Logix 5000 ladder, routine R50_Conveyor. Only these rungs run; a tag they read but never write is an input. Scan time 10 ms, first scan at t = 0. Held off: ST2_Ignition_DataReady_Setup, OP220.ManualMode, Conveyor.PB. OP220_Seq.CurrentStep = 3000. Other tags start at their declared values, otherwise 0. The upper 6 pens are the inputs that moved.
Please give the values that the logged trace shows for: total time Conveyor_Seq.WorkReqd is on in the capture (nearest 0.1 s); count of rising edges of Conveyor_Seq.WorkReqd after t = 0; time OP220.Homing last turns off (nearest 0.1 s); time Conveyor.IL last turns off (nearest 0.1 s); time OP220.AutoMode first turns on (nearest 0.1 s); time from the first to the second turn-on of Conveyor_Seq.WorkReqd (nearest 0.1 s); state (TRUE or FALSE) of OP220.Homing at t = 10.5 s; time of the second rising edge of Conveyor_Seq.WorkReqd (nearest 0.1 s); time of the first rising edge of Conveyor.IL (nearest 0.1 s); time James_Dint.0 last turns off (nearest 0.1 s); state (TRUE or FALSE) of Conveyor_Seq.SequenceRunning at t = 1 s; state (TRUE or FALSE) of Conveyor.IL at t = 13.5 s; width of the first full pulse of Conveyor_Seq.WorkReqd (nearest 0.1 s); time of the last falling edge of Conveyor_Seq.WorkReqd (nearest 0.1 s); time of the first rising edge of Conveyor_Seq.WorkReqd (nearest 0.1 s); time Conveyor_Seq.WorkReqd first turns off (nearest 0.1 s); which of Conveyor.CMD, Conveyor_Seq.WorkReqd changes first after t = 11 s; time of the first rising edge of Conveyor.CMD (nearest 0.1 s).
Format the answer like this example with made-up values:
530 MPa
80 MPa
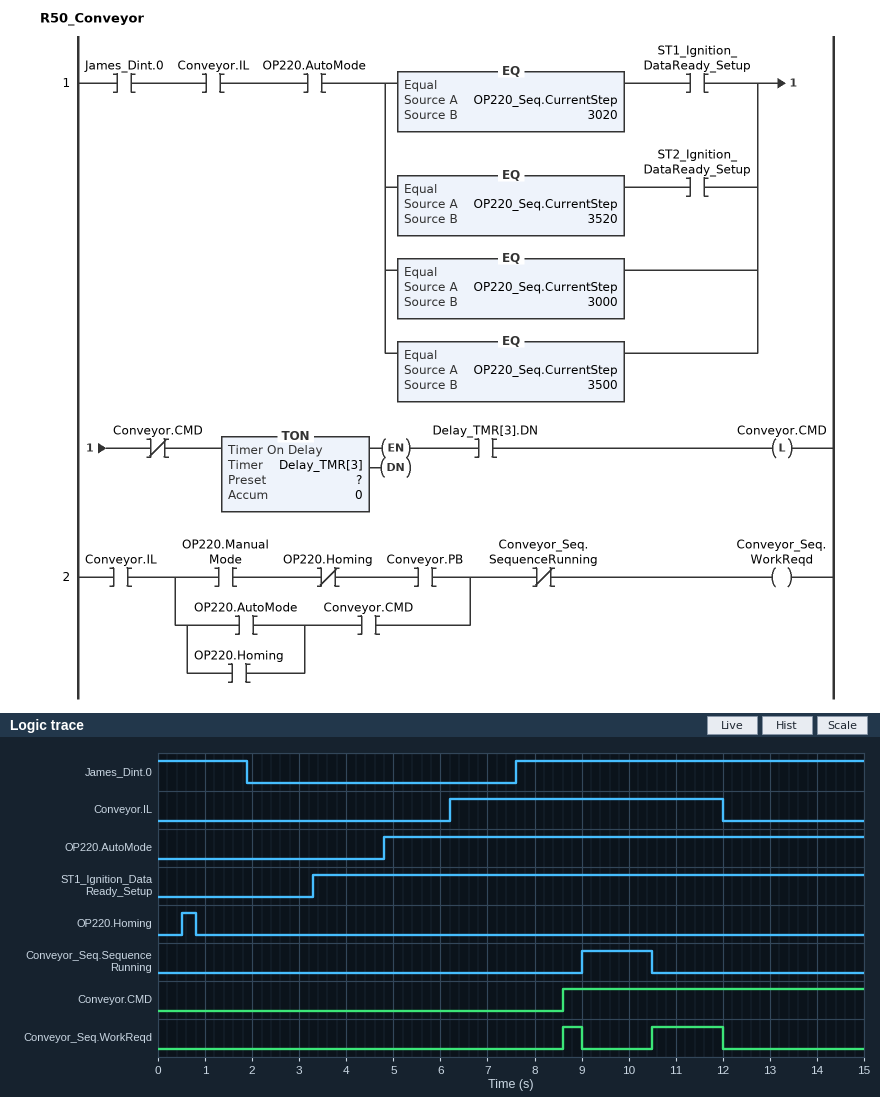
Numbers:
1.9 s
2
0.8 s
12.0 s
4.8 s
1.9 s
FALSE
10.5 s
6.2 s
1.9 s
FALSE
FALSE
0.4 s
12.0 s
8.6 s
9.0 s
Conveyor_Seq.WorkReqd
8.6 s
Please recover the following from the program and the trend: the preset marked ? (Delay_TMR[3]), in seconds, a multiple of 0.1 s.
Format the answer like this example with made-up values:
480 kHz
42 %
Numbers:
1.0 s
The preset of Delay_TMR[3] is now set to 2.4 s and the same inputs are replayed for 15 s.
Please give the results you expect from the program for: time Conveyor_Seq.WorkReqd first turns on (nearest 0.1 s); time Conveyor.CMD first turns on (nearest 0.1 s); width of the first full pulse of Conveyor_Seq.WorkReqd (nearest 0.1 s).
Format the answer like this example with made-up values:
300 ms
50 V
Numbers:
10.5 s
10.0 s
1.5 s
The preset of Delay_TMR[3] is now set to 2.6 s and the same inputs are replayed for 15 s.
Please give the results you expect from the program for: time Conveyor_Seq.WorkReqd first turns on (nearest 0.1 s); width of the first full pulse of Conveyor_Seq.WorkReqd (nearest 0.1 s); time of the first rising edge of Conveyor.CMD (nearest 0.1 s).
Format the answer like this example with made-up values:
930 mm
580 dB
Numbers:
10.5 s
1.5 s
10.2 s
